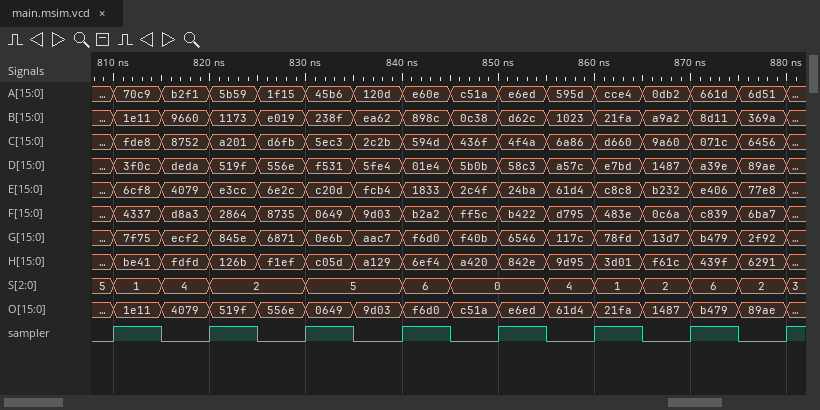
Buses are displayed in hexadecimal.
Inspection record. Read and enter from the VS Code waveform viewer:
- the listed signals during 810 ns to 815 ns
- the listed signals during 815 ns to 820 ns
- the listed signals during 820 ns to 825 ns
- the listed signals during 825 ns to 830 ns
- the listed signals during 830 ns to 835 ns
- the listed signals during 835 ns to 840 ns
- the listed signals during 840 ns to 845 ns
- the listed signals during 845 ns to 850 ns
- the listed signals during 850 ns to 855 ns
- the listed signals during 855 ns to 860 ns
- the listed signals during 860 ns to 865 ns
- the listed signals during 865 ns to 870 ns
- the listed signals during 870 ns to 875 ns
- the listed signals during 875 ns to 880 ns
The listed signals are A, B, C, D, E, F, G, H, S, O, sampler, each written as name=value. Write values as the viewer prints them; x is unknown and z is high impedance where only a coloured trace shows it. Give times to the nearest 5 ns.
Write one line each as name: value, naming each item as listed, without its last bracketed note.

the listed signals during 810 ns to 815 ns: A=70c9, B=1e11, C=fde8, D=3f0c, E=6cf8, F=4337, G=7f75, H=be41, S=1, O=1e11, sampler=1
the listed signals during 815 ns to 820 ns: A=b2f1, B=9660, C=8752, D=deda, E=4079, F=d8a3, G=ecf2, H=fdfd, S=4, O=4079, sampler=0
the listed signals during 820 ns to 825 ns: A=5b59, B=1173, C=a201, D=519f, E=e3cc, F=2864, G=845e, H=126b, S=2, O=519f, sampler=1
the listed signals during 825 ns to 830 ns: A=1f15, B=e019, C=d6fb, D=556e, E=6e2c, F=8735, G=6871, H=f1ef, S=2, O=556e, sampler=0
the listed signals during 830 ns to 835 ns: A=45b6, B=238f, C=5ec3, D=f531, E=c20d, F=0649, G=0e6b, H=c05d, S=5, O=0649, sampler=1
the listed signals during 835 ns to 840 ns: A=120d, B=ea62, C=2c2b, D=5fe4, E=fcb4, F=9d03, G=aac7, H=a129, S=5, O=9d03, sampler=0
the listed signals during 840 ns to 845 ns: A=e60e, B=898c, C=594d, D=01e4, E=1833, F=b2a2, G=f6d0, H=6ef4, S=6, O=f6d0, sampler=1
the listed signals during 845 ns to 850 ns: A=c51a, B=0c38, C=436f, D=5b0b, E=2c4f, F=ff5c, G=f40b, H=a420, S=0, O=c51a, sampler=0
the listed signals during 850 ns to 855 ns: A=e6ed, B=d62c, C=4f4a, D=58c3, E=24ba, F=b422, G=6546, H=842e, S=0, O=e6ed, sampler=1
the listed signals during 855 ns to 860 ns: A=595d, B=1023, C=6a86, D=a57c, E=61d4, F=d795, G=117c, H=9d95, S=4, O=61d4, sampler=0
the listed signals during 860 ns to 865 ns: A=cce4, B=21fa, C=d660, D=e7bd, E=c8c8, F=483e, G=78fd, H=3d01, S=1, O=21fa, sampler=1
the listed signals during 865 ns to 870 ns: A=0db2, B=a9a2, C=9a60, D=1487, E=b232, F=0c6a, G=13d7, H=f61c, S=2, O=1487, sampler=0
the listed signals during 870 ns to 875 ns: A=661d, B=8d11, C=071c, D=a39e, E=e406, F=c839, G=b479, H=439f, S=6, O=b479, sampler=1
the listed signals during 875 ns to 880 ns: A=6d51, B=369a, C=6456, D=89ae, E=77e8, F=6ba7, G=2f92, H=6291, S=2, O=89ae, sampler=0
